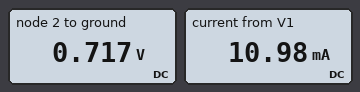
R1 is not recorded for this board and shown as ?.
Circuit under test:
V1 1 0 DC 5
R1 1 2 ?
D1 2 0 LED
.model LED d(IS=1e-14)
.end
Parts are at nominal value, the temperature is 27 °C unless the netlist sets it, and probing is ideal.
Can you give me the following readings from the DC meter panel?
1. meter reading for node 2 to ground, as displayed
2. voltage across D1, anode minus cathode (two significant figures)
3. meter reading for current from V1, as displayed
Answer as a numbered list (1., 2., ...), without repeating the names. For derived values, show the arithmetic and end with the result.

1. 0.717 V
2. 717 mV = 720 mV
3. 10.98 mA
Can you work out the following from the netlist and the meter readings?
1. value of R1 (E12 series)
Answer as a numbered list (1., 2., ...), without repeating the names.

1. 390 Ω
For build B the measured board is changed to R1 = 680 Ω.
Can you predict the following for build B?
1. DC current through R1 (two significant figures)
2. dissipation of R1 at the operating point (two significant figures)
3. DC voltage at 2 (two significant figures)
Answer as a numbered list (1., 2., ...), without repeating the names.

1. 6.3 mA
2. 27 mW
3. 700 mV
